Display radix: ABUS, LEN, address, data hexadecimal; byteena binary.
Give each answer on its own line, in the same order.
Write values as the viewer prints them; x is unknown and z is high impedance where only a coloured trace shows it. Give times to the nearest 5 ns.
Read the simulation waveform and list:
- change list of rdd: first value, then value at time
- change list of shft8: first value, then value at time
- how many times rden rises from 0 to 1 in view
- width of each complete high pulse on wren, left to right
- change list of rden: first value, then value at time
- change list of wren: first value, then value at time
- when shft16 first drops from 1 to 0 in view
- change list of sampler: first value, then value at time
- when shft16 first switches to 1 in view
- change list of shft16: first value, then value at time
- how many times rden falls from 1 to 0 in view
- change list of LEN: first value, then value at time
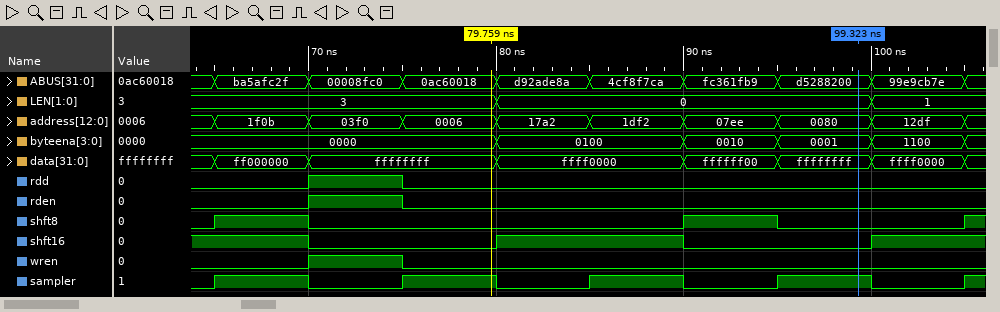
0, 1 at 70 ns, 0 at 75 ns
0, 1 at 65 ns, 0 at 70 ns, 1 at 90 ns, 0 at 95 ns, 1 at 105 ns
1
5 ns
0, 1 at 70 ns, 0 at 75 ns
0, 1 at 70 ns, 0 at 75 ns
70 ns
0, 1 at 65 ns, 0 at 70 ns, 1 at 75 ns, 0 at 80 ns, 1 at 85 ns, 0 at 90 ns, 1 at 95 ns, 0 at 100 ns, 1 at 105 ns
80 ns
1, 0 at 70 ns, 1 at 80 ns, 0 at 90 ns, 1 at 100 ns
1
3, 0 at 80 ns, 1 at 100 ns
